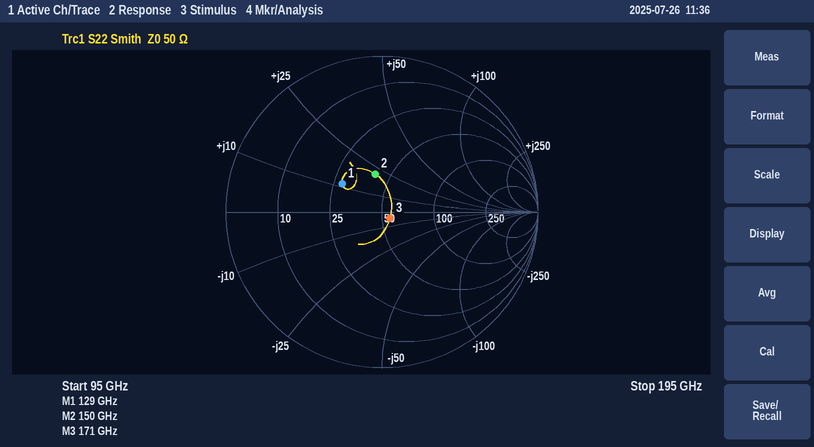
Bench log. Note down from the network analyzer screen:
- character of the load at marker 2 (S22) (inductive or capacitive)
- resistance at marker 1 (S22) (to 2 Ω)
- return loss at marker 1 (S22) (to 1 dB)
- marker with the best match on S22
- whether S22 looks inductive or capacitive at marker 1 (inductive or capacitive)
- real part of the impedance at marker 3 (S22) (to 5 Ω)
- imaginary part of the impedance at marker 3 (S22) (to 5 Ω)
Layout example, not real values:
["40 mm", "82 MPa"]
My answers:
["inductive", "28 Ω", "10 dB", "marker 3", "inductive", "55 Ω", "-5 Ω"]
